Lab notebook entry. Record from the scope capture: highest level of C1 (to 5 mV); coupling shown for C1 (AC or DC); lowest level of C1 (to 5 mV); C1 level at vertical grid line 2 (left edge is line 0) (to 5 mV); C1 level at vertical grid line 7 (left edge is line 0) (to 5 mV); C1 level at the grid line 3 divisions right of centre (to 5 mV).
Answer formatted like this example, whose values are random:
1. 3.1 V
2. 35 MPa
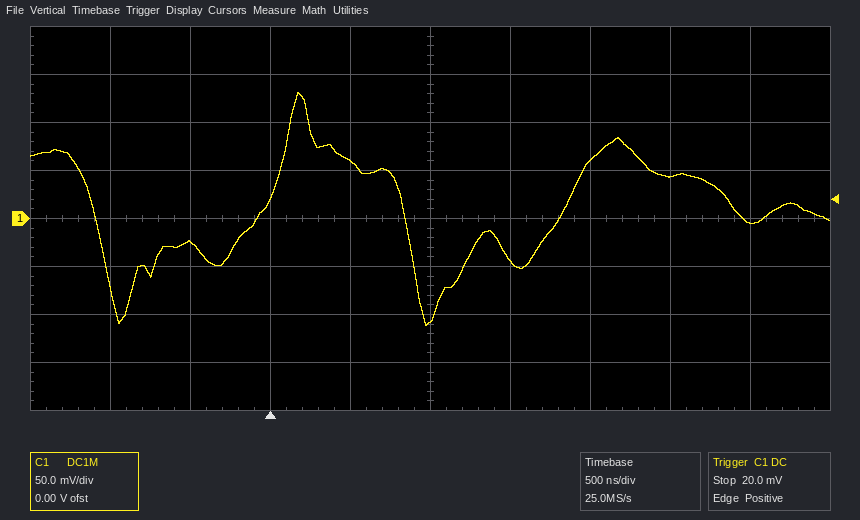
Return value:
1. 130 mV
2. DC
3. -110 mV
4. -25 mV
5. 60 mV
6. 45 mV
